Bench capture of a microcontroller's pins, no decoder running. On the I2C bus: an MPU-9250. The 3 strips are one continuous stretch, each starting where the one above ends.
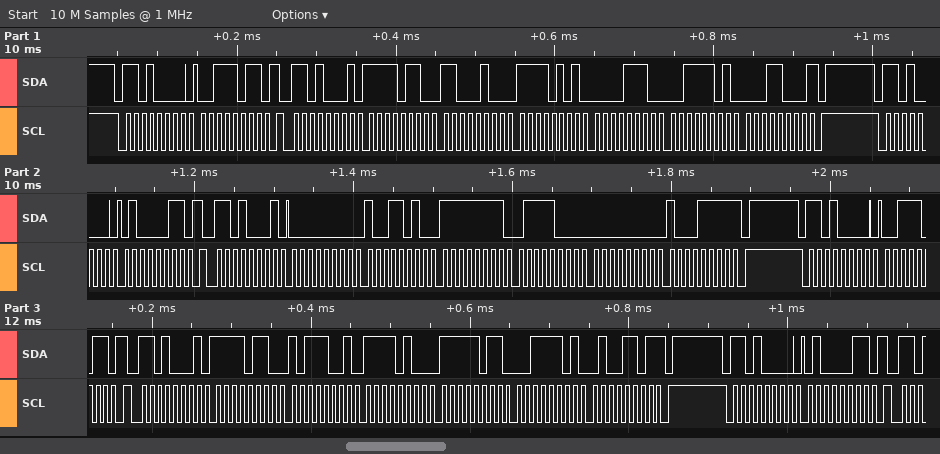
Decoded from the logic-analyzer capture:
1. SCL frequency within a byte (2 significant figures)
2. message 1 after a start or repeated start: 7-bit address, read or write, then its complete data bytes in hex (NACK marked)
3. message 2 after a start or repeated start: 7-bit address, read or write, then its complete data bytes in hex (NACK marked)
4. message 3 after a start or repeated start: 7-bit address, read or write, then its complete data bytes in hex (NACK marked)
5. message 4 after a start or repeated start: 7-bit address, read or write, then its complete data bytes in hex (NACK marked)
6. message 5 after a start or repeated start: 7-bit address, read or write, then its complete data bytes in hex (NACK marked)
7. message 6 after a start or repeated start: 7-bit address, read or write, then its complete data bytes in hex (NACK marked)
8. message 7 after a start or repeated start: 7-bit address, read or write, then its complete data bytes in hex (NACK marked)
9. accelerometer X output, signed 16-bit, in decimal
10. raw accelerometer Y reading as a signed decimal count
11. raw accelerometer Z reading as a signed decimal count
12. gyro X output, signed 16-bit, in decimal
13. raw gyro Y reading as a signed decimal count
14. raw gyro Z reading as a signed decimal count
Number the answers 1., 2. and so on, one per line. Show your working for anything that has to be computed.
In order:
1. 100 kHz
2. 0x68 write: 3B
3. 0x68 read: F6 C4 F5 0E 3D 18 NACK
4. 0x68 write: 43
5. 0x68 read: 00 9A FF 78 00 8F NACK
6. 0x68 write: 3B
7. 0x68 read: F6 B9 F4 FB 3D 4D NACK
8. 0x68 write: 43
9. 0xF6C4 = -2364
10. 0xF50E = -2802
11. 0x3D18 = 15640
12. 0x009A = 154
13. 0xFF78 = -136
14. 0x008F = 143
